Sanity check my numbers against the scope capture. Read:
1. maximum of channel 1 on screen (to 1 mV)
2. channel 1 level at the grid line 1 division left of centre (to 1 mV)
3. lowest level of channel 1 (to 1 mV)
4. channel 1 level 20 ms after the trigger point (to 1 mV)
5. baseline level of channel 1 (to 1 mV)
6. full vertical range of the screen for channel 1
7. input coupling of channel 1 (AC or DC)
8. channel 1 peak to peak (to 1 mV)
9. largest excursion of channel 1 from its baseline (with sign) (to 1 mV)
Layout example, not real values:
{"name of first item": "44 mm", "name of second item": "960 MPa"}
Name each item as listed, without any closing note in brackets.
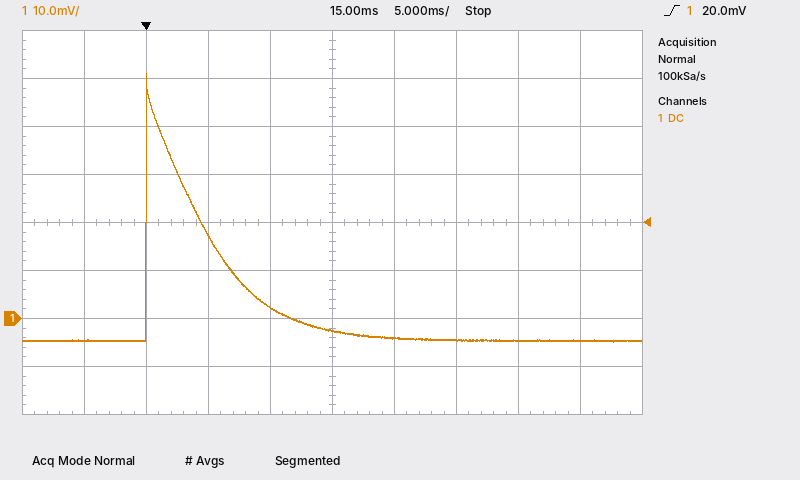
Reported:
{"maximum of channel 1 on screen": "51 mV", "channel 1 level at the grid line 1 division left of centre": "2 mV", "lowest level of channel 1": "-5 mV", "channel 1 level 20 ms after the trigger point": "-4 mV", "baseline level of channel 1": "-5 mV", "full vertical range of the screen for channel 1": "80 mV", "input coupling of channel 1": "DC", "channel 1 peak to peak": "56 mV", "largest excursion of channel 1 from its baseline (with sign)": "+56 mV"}
